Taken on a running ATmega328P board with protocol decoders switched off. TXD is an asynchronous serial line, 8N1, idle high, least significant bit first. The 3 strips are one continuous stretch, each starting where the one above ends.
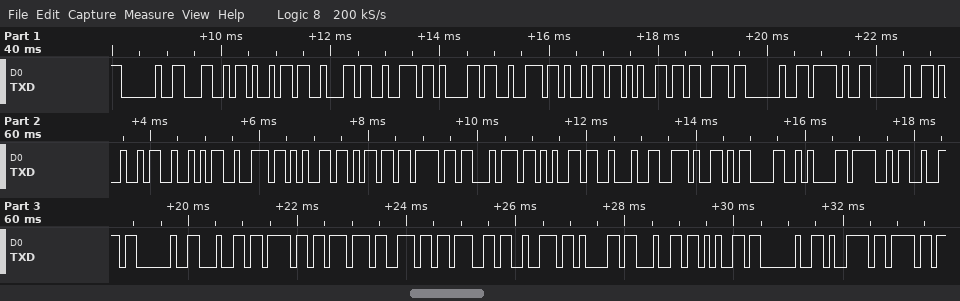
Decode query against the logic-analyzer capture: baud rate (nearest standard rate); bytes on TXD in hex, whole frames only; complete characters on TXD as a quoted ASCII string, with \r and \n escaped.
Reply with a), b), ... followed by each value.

a) 9600 baud
b) 20 4C 69 62 72 61 72 69 65 73 20 2F 20 49 52 72 65 6D 6F 74 65 22 2E 0D 0A 4F 72 20 64 6F 77 6E 67 72 61 64 65 20 79 6F
c) " Libraries / IRremote\".\r\nOr downgrade yo"
